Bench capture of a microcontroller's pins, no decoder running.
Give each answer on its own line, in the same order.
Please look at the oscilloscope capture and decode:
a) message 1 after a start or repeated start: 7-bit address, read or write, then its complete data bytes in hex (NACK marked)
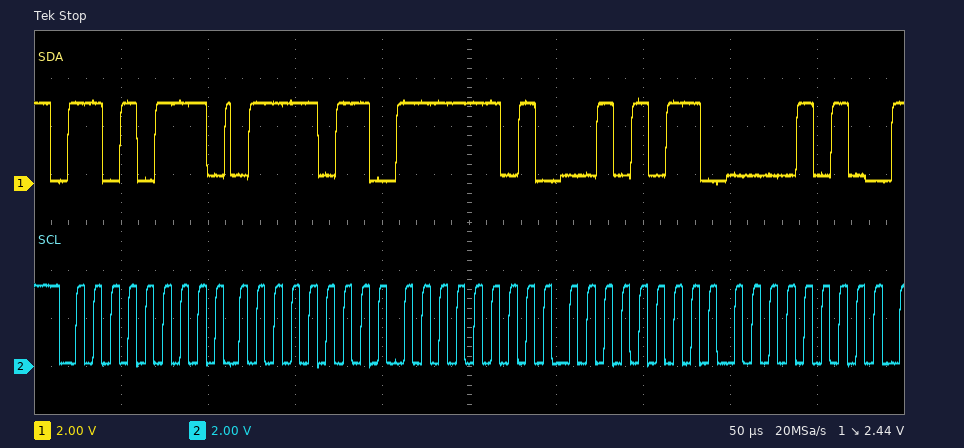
0x6B read: 7B FD 2B 0A
